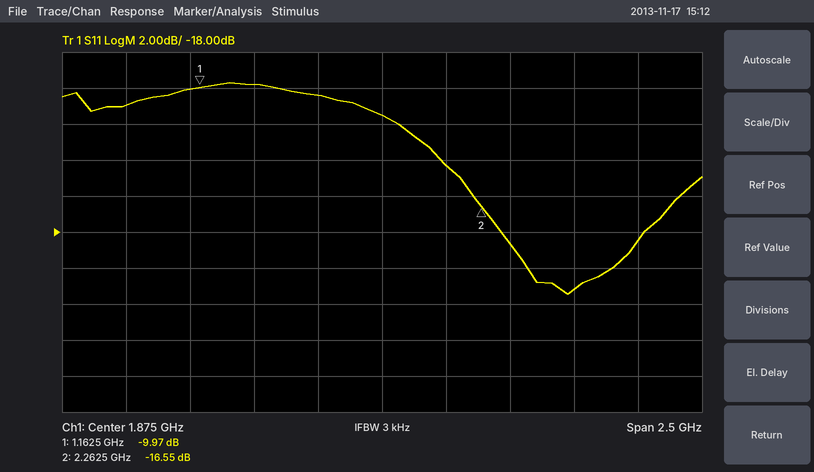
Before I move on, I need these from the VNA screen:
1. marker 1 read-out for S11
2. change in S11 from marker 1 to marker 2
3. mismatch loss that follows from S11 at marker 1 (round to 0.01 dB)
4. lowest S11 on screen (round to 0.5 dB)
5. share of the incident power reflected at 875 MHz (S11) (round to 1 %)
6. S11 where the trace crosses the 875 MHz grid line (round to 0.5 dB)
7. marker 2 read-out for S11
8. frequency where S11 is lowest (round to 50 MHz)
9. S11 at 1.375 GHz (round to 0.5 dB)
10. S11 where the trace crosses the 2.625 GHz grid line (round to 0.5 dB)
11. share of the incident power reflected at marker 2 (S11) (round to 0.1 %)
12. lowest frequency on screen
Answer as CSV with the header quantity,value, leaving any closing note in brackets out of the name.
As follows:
quantity,value
marker 1 read-out for S11,-9.97 dB
change in S11 from marker 1 to marker 2,-6.58 dB
mismatch loss that follows from S11 at marker 1,0.46 dB
lowest S11 on screen,-21.5 dB
share of the incident power reflected at 875 MHz (S11),8 %
S11 where the trace crosses the 875 MHz grid line,-11.0 dB
marker 2 read-out for S11,-16.55 dB
frequency where S11 is lowest,2.60 GHz
S11 at 1.375 GHz,-10.0 dB
S11 where the trace crosses the 2.625 GHz grid line,-21.0 dB
share of the incident power reflected at marker 2 (S11),2.2 %
lowest frequency on screen,625 MHz
